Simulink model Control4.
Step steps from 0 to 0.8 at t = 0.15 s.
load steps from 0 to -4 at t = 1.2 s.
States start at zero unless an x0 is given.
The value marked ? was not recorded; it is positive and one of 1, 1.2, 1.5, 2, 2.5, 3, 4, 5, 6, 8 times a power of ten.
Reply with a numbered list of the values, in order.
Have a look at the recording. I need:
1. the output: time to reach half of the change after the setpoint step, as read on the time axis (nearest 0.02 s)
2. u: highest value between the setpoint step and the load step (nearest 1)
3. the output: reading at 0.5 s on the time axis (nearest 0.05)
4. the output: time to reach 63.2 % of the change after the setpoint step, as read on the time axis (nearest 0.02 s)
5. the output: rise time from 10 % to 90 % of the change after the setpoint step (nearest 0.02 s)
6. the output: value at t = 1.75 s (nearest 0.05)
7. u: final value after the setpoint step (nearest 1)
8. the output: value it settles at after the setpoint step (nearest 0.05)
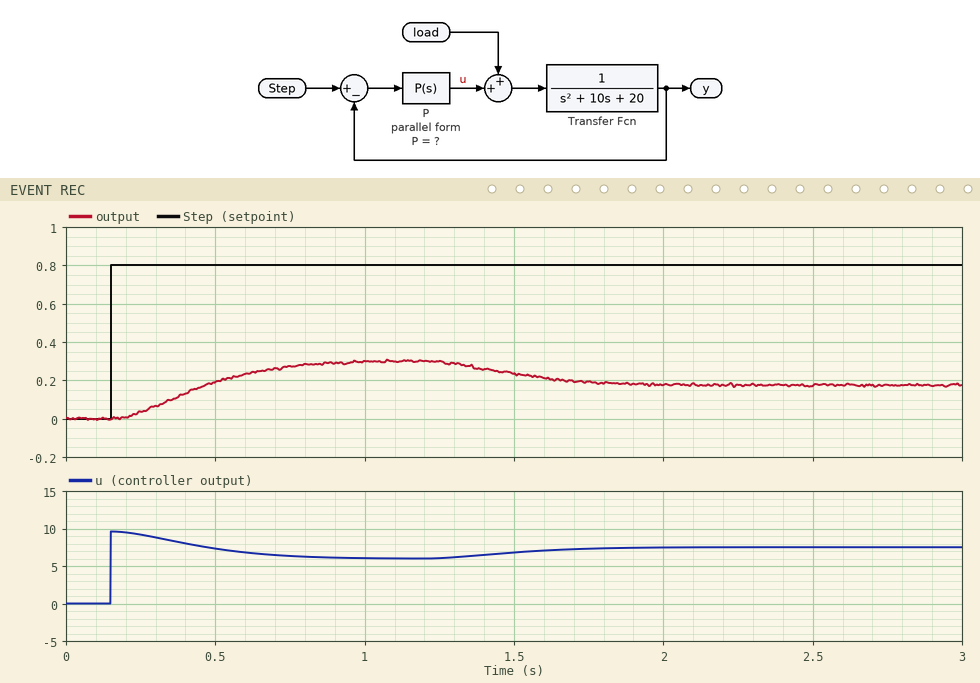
1. 0.42 s
2. 10
3. 0.20
4. 0.50 s
5. 0.50 s
6. 0.20
7. 6
8. 0.30
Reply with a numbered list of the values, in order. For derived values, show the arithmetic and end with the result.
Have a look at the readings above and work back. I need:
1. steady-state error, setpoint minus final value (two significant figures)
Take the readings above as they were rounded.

1. 0.8 - 0.3 = 0.50
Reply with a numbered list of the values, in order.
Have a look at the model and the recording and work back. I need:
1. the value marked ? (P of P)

1. 12
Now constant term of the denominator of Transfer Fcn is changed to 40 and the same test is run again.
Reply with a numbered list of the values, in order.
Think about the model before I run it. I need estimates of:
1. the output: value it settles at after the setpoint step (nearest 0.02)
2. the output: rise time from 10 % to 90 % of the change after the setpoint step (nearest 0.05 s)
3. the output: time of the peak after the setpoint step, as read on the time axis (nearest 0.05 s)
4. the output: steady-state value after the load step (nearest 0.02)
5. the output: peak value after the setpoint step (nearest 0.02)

1. 0.18
2. 0.30 s
3. 0.75 s
4. 0.10
5. 0.20
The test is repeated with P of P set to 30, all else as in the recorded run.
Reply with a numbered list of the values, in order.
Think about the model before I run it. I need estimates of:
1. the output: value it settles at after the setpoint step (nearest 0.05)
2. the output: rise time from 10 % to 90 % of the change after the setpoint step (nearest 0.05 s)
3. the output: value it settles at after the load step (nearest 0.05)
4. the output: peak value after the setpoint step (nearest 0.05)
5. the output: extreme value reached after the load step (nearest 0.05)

1. 0.50
2. 0.30 s
3. 0.40
4. 0.50
5. 0.40
